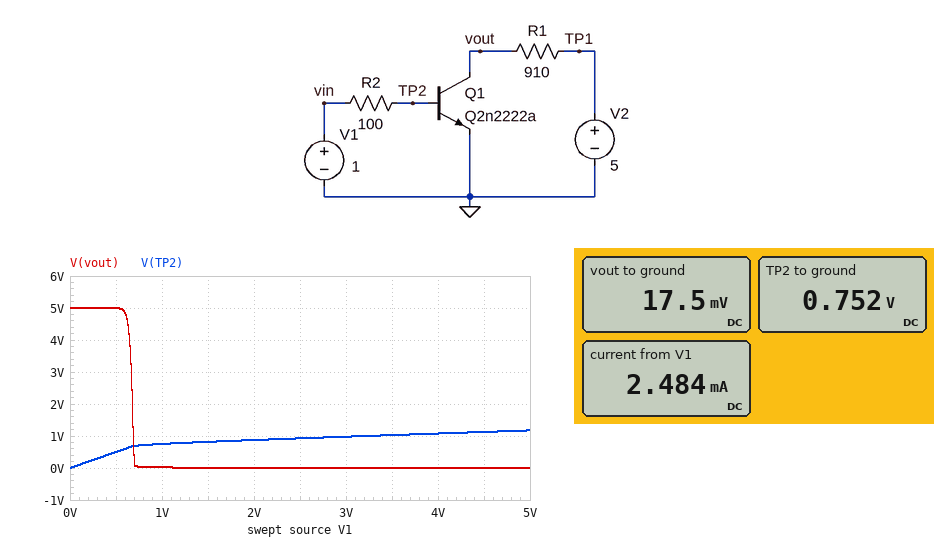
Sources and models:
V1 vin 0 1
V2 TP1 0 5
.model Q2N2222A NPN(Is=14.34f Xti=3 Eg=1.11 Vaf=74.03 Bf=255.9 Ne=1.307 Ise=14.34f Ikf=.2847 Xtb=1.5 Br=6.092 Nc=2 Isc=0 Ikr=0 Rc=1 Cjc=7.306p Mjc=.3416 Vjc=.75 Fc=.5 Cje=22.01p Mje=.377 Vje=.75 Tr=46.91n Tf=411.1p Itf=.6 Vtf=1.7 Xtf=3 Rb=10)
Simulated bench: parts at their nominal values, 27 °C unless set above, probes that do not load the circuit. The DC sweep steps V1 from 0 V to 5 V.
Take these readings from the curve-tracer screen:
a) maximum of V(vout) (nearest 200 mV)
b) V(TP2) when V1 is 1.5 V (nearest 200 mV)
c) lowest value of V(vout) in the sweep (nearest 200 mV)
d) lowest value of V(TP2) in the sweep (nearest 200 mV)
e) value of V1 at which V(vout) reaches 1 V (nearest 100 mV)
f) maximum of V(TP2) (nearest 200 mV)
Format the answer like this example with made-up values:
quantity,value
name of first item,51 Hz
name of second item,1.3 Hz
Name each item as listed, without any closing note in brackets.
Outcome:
quantity,value
maximum of V(vout),5.0 V
V(TP2) when V1 is 1.5 V,800 mV
lowest value of V(vout) in the sweep,0 V
lowest value of V(TP2) in the sweep,0 V
value of V1 at which V(vout) reaches 1 V,700 mV
maximum of V(TP2),1.2 V
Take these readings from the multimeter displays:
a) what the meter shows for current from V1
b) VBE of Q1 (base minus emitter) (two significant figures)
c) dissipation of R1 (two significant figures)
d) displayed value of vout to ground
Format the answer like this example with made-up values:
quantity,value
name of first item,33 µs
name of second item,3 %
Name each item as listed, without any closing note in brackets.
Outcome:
quantity,value
what the meter shows for current from V1,2.484 mA
VBE of Q1 (base minus emitter),750 mV
dissipation of R1,27 mW
displayed value of vout to ground,17.5 mV
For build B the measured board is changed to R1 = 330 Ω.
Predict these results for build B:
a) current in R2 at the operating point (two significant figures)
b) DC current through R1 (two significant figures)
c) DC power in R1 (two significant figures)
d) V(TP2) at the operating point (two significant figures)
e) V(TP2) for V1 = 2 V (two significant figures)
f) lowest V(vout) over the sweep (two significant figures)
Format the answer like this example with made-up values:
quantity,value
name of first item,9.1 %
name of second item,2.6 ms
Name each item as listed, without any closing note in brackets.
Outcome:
quantity,value
current in R2 at the operating point,2.4 mA
DC current through R1,15 mA
DC power in R1,75 mW
V(TP2) at the operating point,760 mV
V(TP2) for V1 = 2 V,880 mV
lowest V(vout) over the sweep,24 mV
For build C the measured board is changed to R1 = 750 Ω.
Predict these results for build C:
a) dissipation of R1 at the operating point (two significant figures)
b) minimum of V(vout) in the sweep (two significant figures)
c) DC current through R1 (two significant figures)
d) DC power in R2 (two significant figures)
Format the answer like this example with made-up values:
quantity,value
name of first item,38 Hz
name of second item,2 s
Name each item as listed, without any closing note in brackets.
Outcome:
quantity,value
dissipation of R1 at the operating point,33 mW
minimum of V(vout) in the sweep,14 mV
DC current through R1,6.6 mA
DC power in R2,610 µW
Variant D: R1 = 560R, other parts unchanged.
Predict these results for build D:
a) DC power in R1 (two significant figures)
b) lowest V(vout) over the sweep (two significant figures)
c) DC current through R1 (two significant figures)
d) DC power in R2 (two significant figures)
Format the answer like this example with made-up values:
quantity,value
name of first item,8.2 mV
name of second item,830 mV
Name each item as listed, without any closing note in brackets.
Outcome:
quantity,value
DC power in R1,44 mW
lowest V(vout) over the sweep,16 mV
DC current through R1,8.9 mA
DC power in R2,600 µW
